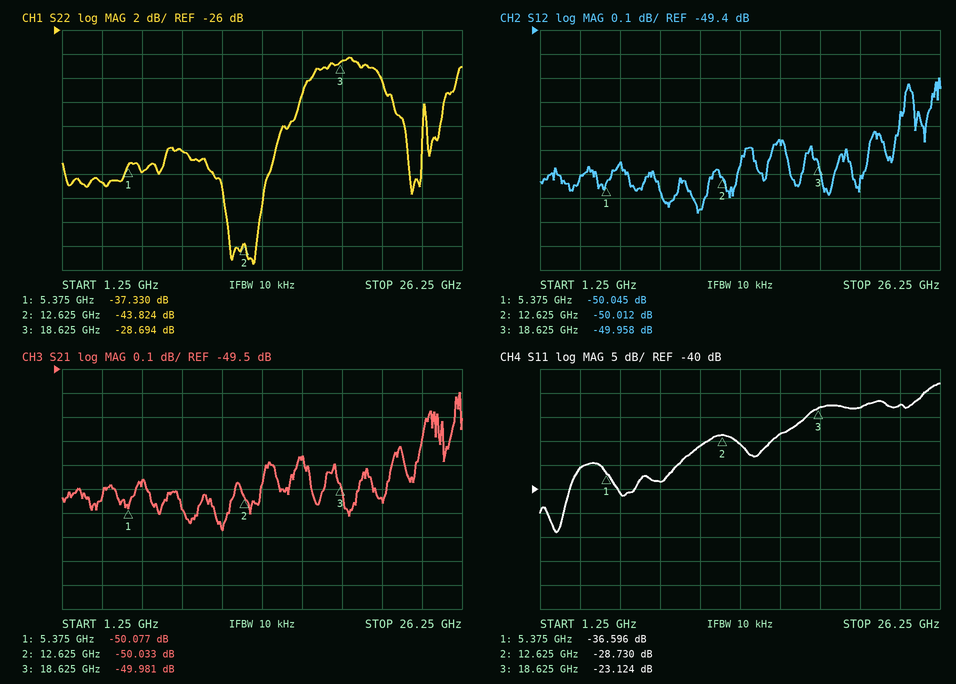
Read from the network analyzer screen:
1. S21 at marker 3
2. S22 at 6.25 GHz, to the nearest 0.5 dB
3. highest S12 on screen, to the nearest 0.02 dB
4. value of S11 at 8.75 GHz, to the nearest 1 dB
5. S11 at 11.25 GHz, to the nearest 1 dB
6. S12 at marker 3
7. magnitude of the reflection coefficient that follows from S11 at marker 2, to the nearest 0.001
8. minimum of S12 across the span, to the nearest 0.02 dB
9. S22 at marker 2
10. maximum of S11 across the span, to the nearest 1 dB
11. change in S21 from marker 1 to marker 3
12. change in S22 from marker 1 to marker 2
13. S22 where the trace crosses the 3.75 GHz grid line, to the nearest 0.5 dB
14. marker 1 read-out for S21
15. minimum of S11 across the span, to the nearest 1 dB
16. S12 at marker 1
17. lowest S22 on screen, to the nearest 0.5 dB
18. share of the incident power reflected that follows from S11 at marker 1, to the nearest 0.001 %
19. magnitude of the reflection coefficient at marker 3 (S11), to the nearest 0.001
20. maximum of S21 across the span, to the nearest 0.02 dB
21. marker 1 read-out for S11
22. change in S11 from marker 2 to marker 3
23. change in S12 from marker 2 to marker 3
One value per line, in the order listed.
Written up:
-49.981 dB
-38.0 dB
-49.60 dB
-38 dB
-31 dB
-49.958 dB
0.037
-50.16 dB
-43.824 dB
-18 dB
0.096 dB
-6.494 dB
-38.5 dB
-50.077 dB
-49 dB
-50.045 dB
-45.5 dB
0.022 %
0.070
-49.60 dB
-36.596 dB
5.606 dB
0.054 dB
